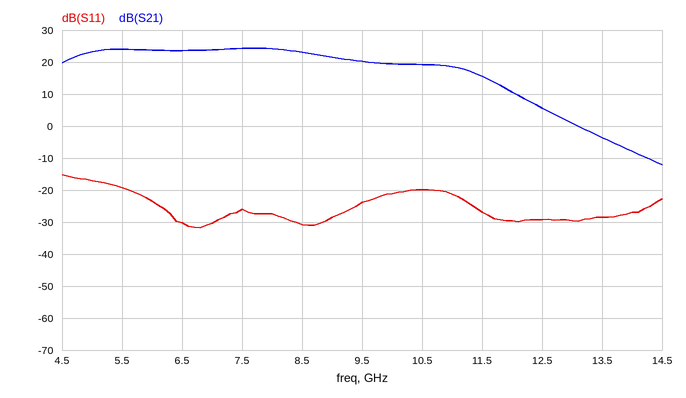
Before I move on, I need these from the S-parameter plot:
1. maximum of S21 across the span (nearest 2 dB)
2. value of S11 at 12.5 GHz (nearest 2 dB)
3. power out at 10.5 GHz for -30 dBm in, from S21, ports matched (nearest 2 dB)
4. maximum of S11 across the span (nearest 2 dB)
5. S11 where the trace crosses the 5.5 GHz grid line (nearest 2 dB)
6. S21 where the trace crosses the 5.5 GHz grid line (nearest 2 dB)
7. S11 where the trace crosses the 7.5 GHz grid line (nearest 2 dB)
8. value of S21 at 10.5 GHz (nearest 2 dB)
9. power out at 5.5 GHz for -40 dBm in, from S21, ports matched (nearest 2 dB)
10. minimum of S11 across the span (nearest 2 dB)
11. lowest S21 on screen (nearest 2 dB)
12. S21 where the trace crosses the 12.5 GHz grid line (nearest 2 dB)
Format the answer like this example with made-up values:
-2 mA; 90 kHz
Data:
24 dB; -30 dB; -10 dBm; -16 dB; -20 dB; 24 dB; -26 dB; 20 dB; -16 dBm; -32 dB; -12 dB; 6 dB
